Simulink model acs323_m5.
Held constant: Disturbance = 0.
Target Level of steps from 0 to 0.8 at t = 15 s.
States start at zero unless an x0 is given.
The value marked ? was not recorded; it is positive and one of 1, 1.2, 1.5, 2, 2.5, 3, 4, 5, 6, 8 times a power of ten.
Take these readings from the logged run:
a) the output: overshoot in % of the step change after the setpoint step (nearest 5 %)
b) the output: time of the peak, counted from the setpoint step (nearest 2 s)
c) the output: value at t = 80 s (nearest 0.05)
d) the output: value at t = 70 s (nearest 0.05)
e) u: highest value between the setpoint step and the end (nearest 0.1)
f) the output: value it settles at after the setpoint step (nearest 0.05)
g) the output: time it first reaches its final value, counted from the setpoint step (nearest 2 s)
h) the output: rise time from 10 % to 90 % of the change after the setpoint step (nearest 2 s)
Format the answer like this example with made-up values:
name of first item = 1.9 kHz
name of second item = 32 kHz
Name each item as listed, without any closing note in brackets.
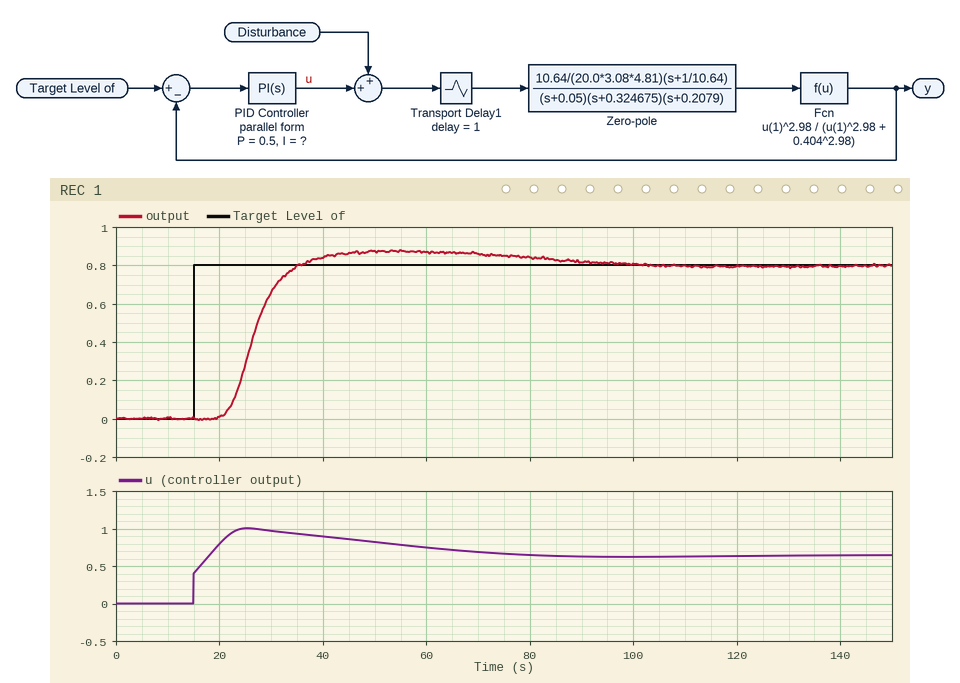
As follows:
the output: overshoot in % of the step change after the setpoint step = 10 %
the output: time of the peak, counted from the setpoint step = 40 s
the output: value at t = 80 s = 0.85
the output: value at t = 70 s = 0.85
u: highest value between the setpoint step and the end = 1.0
the output: value it settles at after the setpoint step = 0.80
the output: time it first reaches its final value, counted from the setpoint step = 20 s
the output: rise time from 10 % to 90 % of the change after the setpoint step = 10 s
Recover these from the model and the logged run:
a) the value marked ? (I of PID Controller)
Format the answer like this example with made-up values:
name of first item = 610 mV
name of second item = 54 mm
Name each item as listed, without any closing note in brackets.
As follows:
the value marked ? = 0.1
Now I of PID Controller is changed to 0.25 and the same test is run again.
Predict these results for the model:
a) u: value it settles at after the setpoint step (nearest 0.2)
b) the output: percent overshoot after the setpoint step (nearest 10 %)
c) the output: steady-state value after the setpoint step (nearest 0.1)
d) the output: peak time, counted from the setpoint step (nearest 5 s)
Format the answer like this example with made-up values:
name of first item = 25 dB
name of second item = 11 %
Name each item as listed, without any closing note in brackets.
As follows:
u: value it settles at after the setpoint step = 0.6
the output: percent overshoot after the setpoint step = 20 %
the output: steady-state value after the setpoint step = 0.8
the output: peak time, counted from the setpoint step = 25 s
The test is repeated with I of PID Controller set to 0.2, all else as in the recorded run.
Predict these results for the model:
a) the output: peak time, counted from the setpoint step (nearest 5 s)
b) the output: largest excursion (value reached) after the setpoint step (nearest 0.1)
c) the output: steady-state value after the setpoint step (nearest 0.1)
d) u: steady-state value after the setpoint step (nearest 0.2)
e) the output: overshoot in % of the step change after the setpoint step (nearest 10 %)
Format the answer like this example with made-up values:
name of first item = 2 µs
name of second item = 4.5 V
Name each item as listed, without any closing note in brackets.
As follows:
the output: peak time, counted from the setpoint step = 30 s
the output: largest excursion (value reached) after the setpoint step = 0.9
the output: steady-state value after the setpoint step = 0.8
u: steady-state value after the setpoint step = 0.6
the output: overshoot in % of the step change after the setpoint step = 20 %
